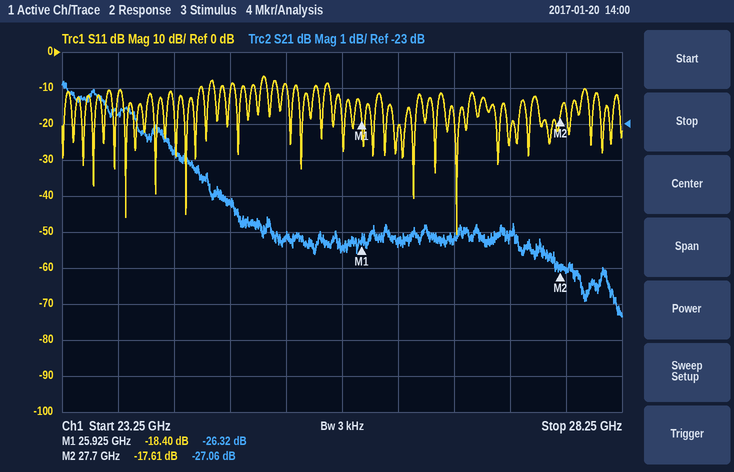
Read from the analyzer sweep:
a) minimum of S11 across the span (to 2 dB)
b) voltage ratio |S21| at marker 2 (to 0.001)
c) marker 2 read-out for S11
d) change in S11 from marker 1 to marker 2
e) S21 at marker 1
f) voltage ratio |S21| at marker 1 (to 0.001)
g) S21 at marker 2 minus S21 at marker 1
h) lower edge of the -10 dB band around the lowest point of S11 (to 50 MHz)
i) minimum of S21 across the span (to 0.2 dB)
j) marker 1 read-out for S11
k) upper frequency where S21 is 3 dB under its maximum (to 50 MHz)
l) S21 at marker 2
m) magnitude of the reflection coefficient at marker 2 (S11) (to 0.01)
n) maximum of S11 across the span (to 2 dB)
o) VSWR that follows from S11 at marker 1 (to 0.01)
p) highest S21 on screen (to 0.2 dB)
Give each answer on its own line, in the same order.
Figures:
-50 dB
0.044
-17.61 dB
0.79 dB
-26.32 dB
0.048
-0.74 dB
25.65 GHz
-28.4 dB
-18.40 dB
24.55 GHz
-27.06 dB
0.13
-6 dB
1.27
-21.8 dB
